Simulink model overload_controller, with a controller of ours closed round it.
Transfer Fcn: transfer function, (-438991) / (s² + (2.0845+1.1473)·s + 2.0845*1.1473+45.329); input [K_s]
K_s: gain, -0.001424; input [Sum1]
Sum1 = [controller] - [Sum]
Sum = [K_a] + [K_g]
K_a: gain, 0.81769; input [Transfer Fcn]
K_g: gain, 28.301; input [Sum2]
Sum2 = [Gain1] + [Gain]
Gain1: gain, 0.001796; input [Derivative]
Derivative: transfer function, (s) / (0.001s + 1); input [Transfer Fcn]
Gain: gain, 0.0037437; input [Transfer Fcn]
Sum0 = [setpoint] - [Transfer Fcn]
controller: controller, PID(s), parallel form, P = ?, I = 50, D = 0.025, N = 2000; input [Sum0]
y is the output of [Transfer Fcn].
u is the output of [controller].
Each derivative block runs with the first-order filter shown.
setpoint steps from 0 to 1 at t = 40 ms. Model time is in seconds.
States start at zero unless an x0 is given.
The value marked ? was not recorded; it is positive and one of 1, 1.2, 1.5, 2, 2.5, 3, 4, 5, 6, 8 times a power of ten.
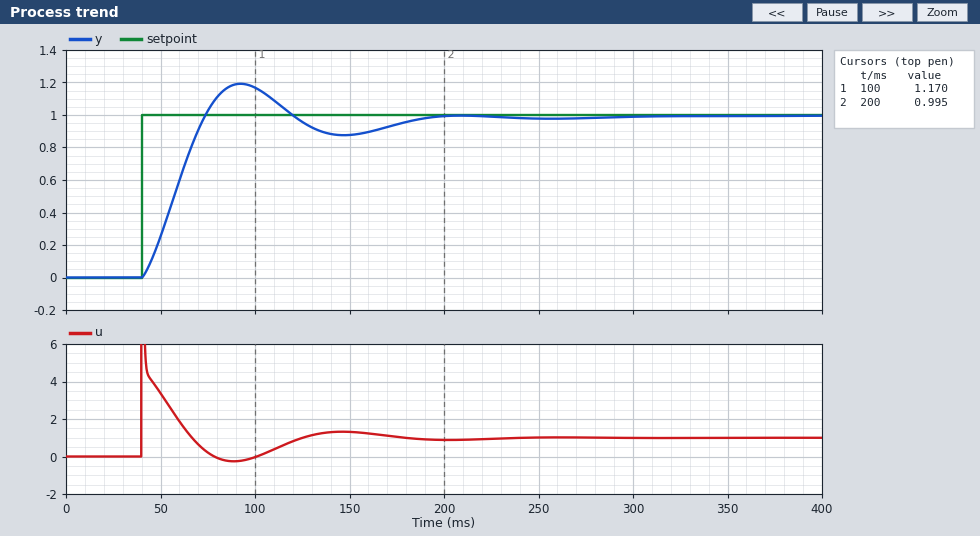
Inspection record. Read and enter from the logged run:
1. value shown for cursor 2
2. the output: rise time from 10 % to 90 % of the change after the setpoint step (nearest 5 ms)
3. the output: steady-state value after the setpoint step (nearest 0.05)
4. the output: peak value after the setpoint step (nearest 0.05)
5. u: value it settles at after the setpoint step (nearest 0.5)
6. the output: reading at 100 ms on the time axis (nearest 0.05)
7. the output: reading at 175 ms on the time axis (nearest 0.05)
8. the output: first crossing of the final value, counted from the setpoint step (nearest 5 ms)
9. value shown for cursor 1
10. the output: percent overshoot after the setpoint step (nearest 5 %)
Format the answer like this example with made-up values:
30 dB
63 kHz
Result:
0.995
25 ms
1.00
1.20
1.0
1.15
0.95
35 ms
1.170
20 %
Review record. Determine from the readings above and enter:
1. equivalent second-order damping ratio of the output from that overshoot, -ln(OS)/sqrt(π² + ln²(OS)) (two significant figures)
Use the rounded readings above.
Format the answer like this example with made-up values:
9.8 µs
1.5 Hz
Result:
0.46
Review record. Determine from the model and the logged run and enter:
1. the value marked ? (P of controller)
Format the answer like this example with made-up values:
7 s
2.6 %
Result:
5
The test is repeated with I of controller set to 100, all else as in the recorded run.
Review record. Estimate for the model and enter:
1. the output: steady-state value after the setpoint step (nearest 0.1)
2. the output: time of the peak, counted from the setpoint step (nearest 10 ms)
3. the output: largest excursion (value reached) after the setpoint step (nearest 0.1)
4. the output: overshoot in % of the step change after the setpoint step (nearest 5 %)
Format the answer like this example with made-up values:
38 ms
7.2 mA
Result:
1.0
50 ms
1.3
35 %
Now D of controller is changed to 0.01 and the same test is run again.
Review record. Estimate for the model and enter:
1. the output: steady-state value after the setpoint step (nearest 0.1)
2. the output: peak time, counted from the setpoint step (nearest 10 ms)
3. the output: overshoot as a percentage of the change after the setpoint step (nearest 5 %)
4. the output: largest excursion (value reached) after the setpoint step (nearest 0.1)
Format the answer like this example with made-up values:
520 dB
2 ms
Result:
1.0
50 ms
30 %
1.3
